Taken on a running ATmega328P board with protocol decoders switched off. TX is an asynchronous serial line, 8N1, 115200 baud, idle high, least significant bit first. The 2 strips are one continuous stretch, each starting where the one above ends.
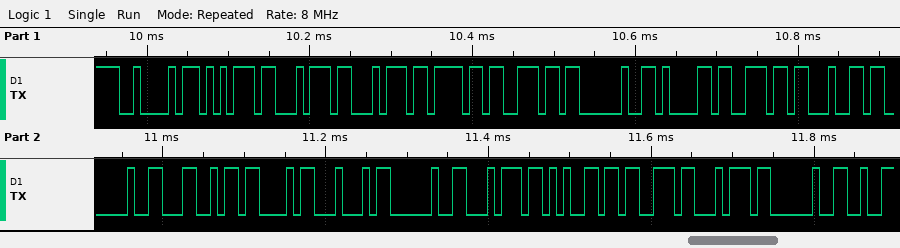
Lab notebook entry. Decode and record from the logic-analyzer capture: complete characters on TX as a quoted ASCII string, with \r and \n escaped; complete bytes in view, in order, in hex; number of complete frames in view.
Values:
"Button and LCD test "
42 75 74 74 6F 6E 20 61 6E 64 20 4C 43 44 20 74 65 73 74 20
20
